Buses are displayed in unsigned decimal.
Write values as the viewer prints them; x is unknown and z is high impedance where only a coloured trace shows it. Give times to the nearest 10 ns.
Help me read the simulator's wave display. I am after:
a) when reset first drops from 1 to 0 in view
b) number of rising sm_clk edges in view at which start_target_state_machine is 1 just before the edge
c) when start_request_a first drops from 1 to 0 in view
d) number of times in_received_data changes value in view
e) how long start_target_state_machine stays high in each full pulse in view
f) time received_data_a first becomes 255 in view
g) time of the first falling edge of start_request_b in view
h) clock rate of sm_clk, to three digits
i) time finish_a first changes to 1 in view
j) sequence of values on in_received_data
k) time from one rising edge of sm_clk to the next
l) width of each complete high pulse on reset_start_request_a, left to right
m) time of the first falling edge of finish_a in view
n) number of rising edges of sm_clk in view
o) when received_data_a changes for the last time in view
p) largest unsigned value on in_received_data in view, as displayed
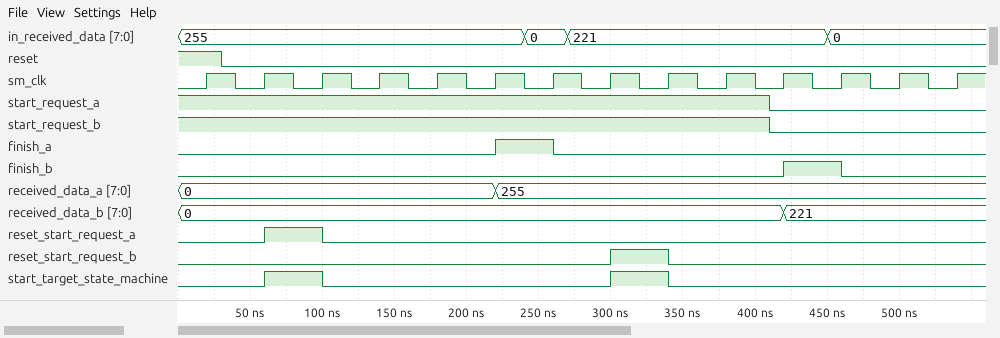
30 ns
2
410 ns
3
40 ns, 40 ns
220 ns
410 ns
25.0 MHz
220 ns
255, 0, 221, 0
40 ns
40 ns
260 ns
14
220 ns
255
